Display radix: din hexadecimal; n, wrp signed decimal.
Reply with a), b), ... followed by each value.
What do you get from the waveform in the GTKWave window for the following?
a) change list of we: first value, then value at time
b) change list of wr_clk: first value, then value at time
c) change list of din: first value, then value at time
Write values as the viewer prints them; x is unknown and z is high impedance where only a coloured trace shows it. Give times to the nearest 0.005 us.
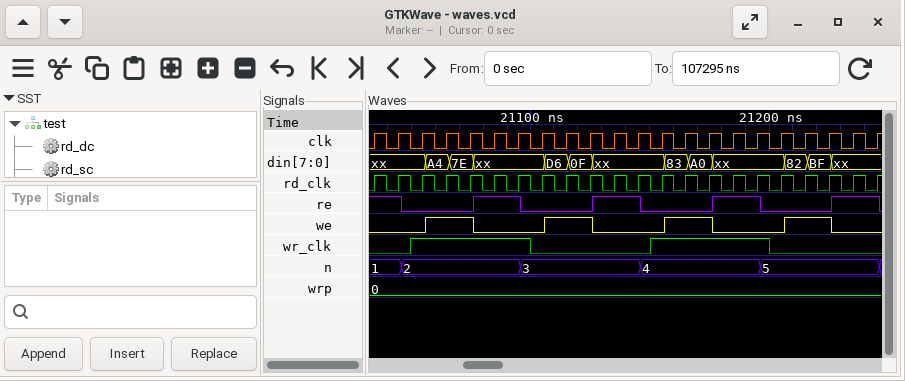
a) 0, 1 at 21.055 us, 0 at 21.075 us, 1 at 21.105 us, 0 at 21.125 us, 1 at 21.155 us, 0 at 21.175 us, 1 at 21.205 us, 0 at 21.225 us
b) 0, 1 at 21.05 us, 0 at 21.1 us, 1 at 21.15 us, 0 at 21.2 us
c) xx, A4 at 21.055 us, 7E at 21.065 us, xx at 21.075 us, D6 at 21.105 us, 0F at 21.115 us, xx at 21.125 us, 83 at 21.155 us, A0 at 21.165 us, xx at 21.175 us, 82 at 21.205 us, BF at 21.215 us, xx at 21.225 us
